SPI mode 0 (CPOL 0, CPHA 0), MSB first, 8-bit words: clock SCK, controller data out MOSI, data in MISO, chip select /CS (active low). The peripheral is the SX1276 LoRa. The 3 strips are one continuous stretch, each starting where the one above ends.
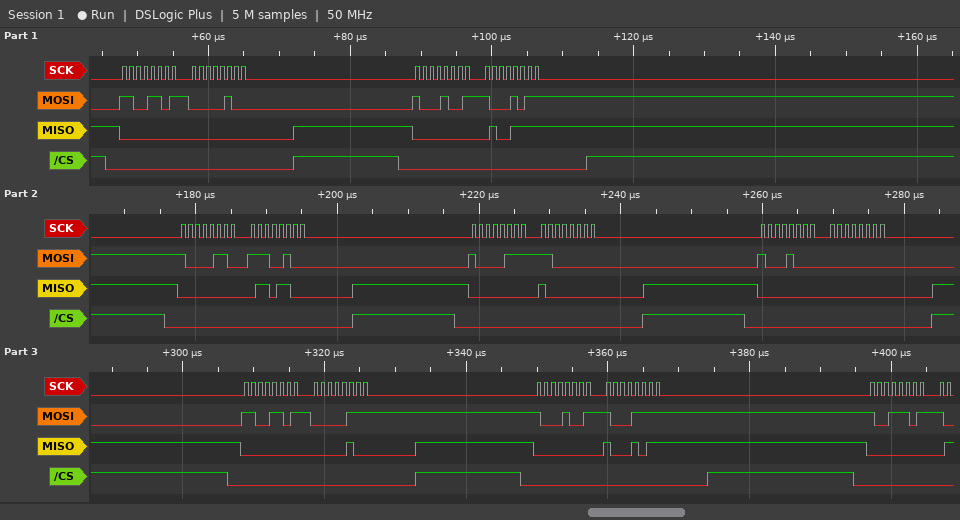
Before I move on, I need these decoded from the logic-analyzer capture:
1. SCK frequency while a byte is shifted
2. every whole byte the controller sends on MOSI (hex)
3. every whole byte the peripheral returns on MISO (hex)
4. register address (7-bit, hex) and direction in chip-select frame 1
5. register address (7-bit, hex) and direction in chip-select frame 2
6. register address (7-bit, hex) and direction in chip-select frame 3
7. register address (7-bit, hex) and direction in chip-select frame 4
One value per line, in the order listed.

1 MHz
CD 04 89 8B 86 E4 87 C0 88 00 CD 07 89 8F 9D
00 00 00 4F 00 6C 00 80 00 00 00 04 00 8B 00
0x4D write
0x09 write
0x06 write
0x07 write
